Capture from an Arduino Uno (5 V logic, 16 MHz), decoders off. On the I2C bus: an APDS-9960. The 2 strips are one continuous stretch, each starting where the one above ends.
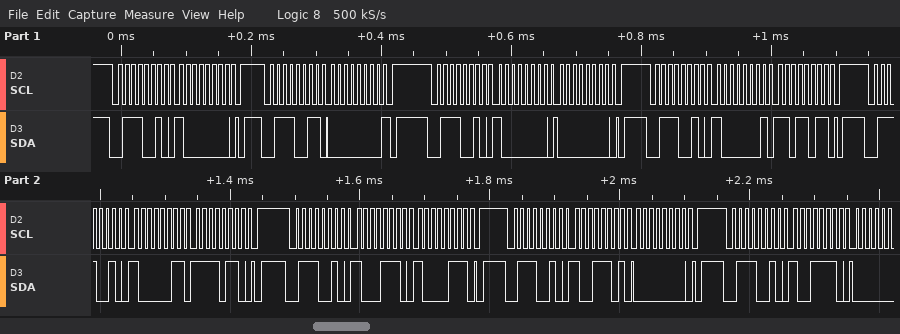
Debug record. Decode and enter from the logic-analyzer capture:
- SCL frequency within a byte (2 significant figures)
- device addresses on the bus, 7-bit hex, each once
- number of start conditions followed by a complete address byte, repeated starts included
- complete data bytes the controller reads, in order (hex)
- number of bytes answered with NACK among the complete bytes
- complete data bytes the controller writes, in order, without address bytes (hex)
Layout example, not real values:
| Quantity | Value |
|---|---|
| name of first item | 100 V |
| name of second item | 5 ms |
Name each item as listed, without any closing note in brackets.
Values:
| Quantity | Value |
|---|---|
| SCL frequency within a byte | 100 kHz |
| device addresses on the bus, 7-bit hex, each once | 0x39 |
| number of start conditions followed by a complete address byte, repeated starts included | 8 |
| complete data bytes the controller reads, in order | 00 |
| number of bytes answered with NACK among the complete bytes | 1 |
| complete data bytes the controller writes, in order, without address bytes | 80 80 00 81 DB 83 F6 8E 87 9D 00 9E |
